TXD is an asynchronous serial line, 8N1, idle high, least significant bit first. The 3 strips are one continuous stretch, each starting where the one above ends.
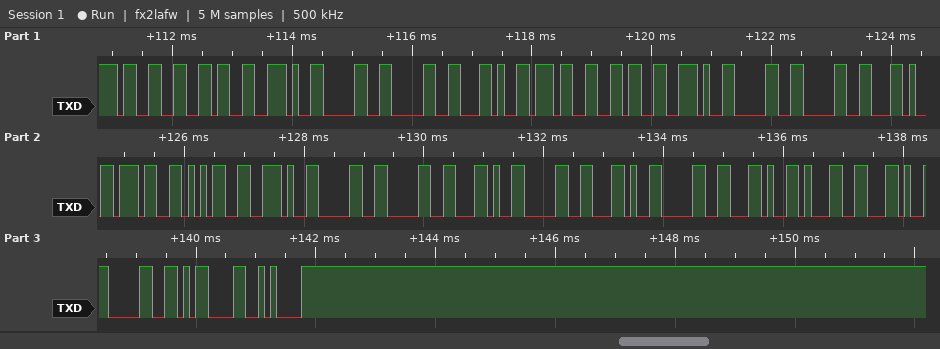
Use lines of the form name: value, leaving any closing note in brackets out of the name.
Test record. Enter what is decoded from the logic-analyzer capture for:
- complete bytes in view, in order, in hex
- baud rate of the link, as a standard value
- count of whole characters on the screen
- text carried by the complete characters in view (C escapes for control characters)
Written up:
complete bytes in view, in order, in hex: 0x33 0x36 0x2E 0x30 0x30 0x2C 0x37 0x36 0x2E 0x30 0x30 0x2C 0x37 0x35 0x2E 0x30 0x30 0x2C 0x30 0x2C 0x30 0x2C 0x31 0x2C 0x30 0x0D 0x0A
baud rate of the link, as a standard value: 9600 baud
count of whole characters on the screen: 27
text carried by the complete characters in view: "36.00,76.00,75.00,0,0,1,0\r\n"
